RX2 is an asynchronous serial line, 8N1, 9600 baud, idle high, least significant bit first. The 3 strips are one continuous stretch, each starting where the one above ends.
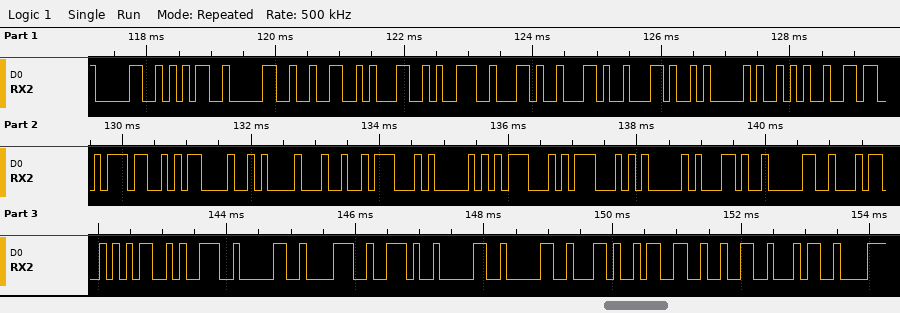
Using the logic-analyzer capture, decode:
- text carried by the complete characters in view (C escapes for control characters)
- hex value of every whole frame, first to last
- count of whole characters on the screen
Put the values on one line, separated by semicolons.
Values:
"050219,,,A*67\r\n$GPGGA,045908.00,324"; 0x30 0x35 0x30 0x32 0x31 0x39 0x2C 0x2C 0x2C 0x41 0x2A 0x36 0x37 0x0D 0x0A 0x24 0x47 0x50 0x47 0x47 0x41 0x2C 0x30 0x34 0x35 0x39 0x30 0x38 0x2E 0x30 0x30 0x2C 0x33 0x32 0x34; 35
